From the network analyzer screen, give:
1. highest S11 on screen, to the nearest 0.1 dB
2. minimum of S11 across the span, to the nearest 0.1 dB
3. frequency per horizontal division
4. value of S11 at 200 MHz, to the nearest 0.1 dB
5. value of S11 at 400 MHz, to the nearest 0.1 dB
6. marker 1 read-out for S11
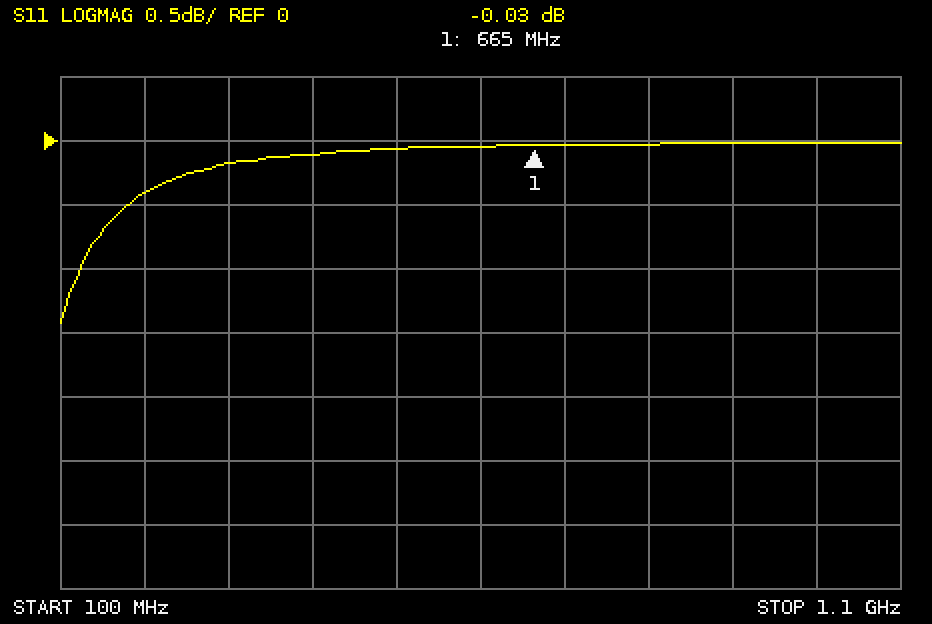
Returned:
0.0 dB
-1.4 dB
100 MHz
-0.4 dB
-0.1 dB
-0.03 dB
